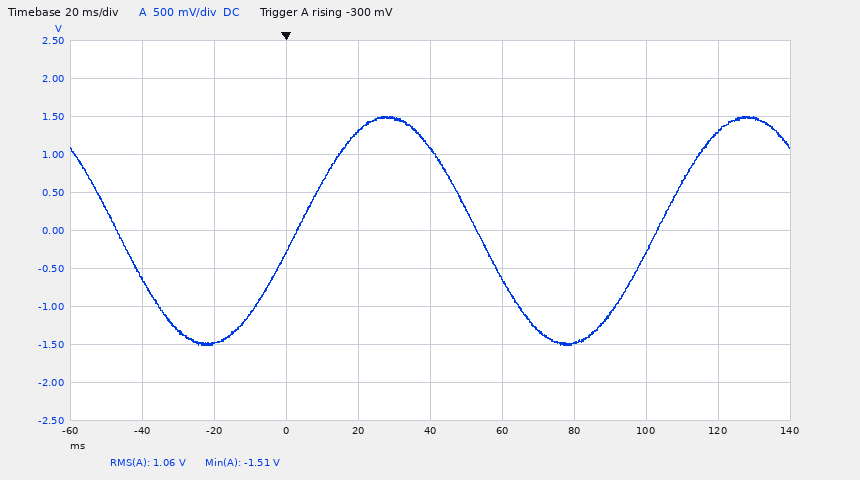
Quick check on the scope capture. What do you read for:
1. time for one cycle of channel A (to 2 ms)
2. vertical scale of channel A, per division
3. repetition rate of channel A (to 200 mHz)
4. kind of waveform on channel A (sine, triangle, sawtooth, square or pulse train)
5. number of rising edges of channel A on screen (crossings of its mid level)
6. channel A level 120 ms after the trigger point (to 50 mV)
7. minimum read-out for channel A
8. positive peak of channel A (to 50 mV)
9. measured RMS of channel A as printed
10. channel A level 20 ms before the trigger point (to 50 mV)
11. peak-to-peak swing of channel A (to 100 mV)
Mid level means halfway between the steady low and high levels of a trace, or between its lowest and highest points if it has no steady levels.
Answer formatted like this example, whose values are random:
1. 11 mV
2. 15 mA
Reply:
1. 100 ms
2. 500 mV
3. 10.0 Hz
4. sine
5. 2
6. 1.30 V
7. -1.51 V
8. 1.50 V
9. 1.06 V
10. -1.50 V
11. 3.00 V
